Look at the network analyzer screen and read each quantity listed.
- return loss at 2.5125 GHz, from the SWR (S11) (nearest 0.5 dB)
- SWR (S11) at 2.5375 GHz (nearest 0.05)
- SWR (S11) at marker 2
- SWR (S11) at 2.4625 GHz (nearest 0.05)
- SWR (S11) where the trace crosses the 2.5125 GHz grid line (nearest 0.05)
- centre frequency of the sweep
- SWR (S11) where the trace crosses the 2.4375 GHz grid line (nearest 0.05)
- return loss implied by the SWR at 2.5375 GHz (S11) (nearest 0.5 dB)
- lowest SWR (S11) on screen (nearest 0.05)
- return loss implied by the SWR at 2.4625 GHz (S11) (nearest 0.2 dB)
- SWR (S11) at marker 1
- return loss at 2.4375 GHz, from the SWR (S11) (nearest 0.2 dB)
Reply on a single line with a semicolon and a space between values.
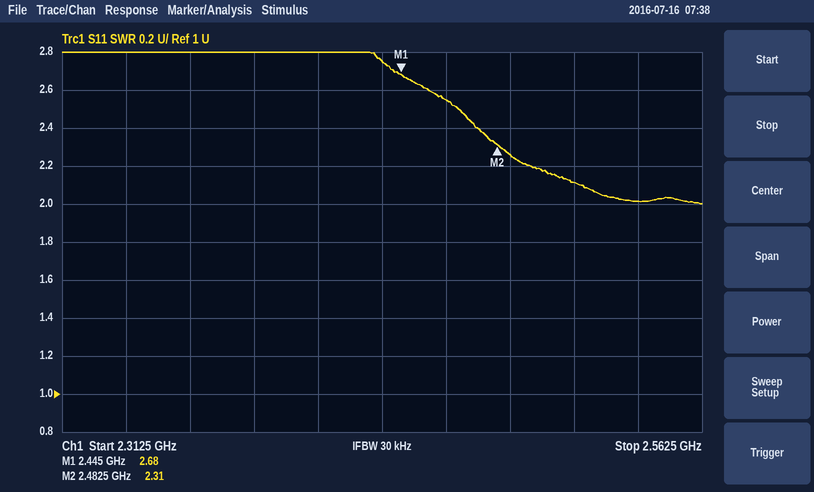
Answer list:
9.0 dB; 2.00; 2.31; 2.55; 2.10; 2.4375 GHz; 2.75; 9.5 dB; 2.00; 7.2 dB; 2.68; 6.6 dB
